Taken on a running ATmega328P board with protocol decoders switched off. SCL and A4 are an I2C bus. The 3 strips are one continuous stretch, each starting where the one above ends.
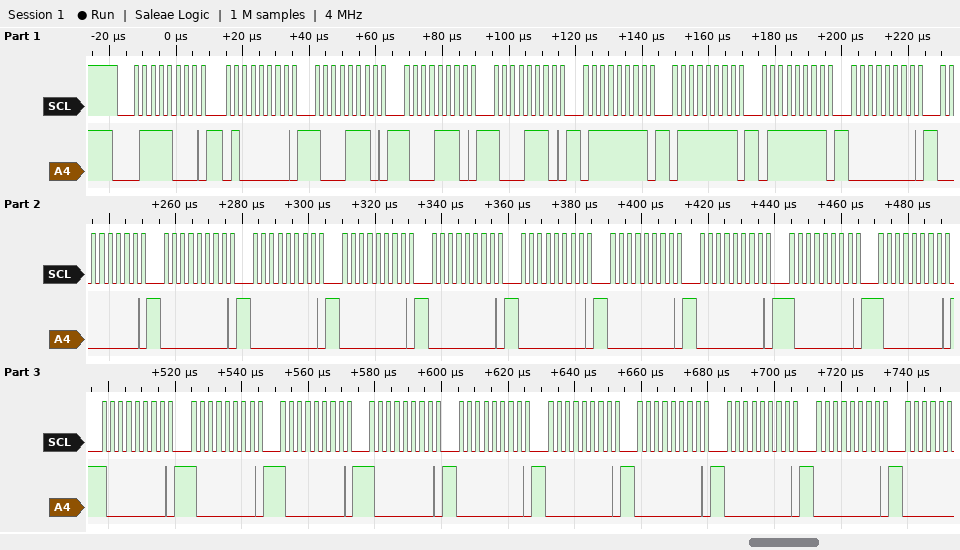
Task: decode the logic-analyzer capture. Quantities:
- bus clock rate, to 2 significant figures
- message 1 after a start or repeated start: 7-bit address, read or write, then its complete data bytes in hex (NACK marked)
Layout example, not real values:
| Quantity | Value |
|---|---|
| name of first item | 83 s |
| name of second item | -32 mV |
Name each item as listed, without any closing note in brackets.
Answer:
| Quantity | Value |
|---|---|
| bus clock rate, to 2 significant figures | 400 kHz |
| message 1 after a start or repeated start: 7-bit address, read or write, then its complete data bytes in hex | 0x3C write: 40 8E 8E 8E 7F 7F 7F 00 00 00 00 00 00 00 00 00 80 80 80 80 80 80 00 00 00 00 00 |
